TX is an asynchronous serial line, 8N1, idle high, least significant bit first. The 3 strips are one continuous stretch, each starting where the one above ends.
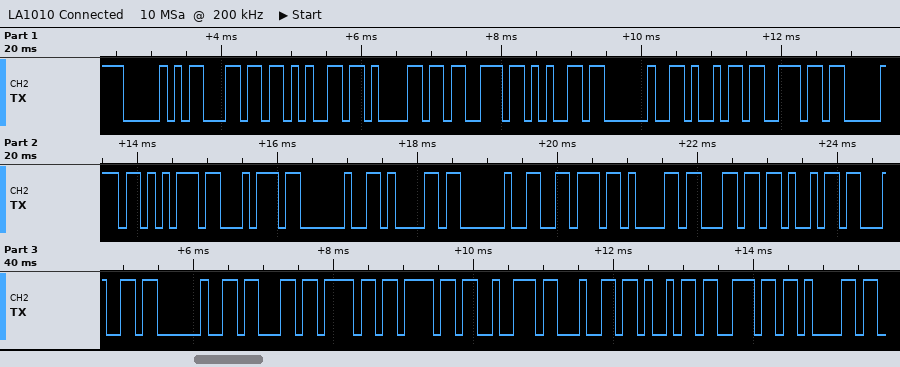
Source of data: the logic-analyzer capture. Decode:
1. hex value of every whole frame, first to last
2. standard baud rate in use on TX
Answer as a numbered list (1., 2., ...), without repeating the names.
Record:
1. 50 6C 65 61 73 65 20 69 6E 70 75 74 20 61 20 76 61 6C 69 64 20 63 6F 6F 72 64 69 6E 61
2. 9600 baud
